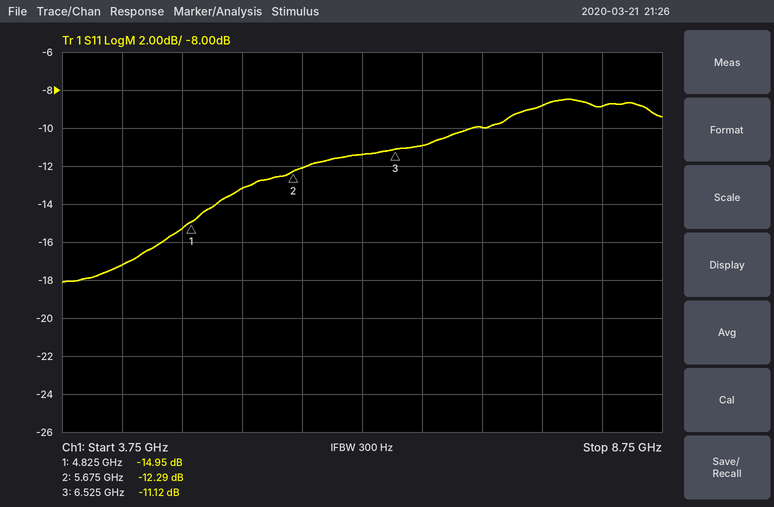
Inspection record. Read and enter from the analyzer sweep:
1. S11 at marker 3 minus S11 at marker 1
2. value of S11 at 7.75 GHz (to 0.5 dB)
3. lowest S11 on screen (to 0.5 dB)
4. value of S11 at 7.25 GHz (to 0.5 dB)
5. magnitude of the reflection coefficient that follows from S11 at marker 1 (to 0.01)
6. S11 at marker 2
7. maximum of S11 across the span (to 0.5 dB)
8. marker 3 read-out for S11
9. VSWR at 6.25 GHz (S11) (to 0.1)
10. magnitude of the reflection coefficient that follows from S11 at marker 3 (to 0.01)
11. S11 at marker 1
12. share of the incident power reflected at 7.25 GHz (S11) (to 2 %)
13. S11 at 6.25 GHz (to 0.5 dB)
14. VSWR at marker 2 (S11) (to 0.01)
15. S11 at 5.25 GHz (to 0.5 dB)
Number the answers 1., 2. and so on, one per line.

1. 3.83 dB
2. -9.0 dB
3. -18.0 dB
4. -10.0 dB
5. 0.18
6. -12.29 dB
7. -8.5 dB
8. -11.12 dB
9. 1.7
10. 0.28
11. -14.95 dB
12. 10 %
13. -11.5 dB
14. 1.64
15. -13.0 dB
